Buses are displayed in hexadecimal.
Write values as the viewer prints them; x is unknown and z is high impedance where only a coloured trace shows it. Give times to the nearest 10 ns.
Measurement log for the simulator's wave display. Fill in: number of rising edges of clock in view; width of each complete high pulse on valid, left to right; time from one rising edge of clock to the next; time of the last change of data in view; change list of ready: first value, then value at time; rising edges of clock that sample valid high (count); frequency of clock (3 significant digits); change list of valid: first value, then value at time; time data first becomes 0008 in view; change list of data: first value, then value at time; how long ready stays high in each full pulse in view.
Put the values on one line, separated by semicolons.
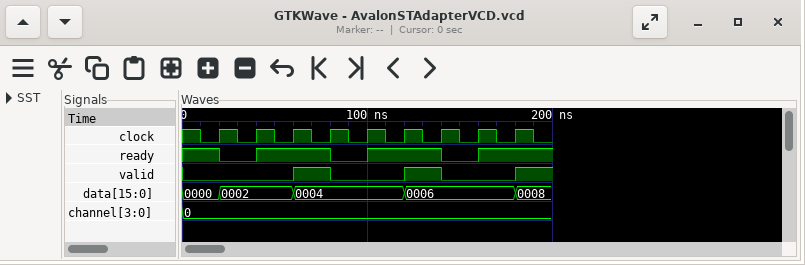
9; 20 ns, 20 ns; 20 ns; 180 ns; 1, 0 at 20 ns, 1 at 40 ns, 0 at 80 ns, 1 at 100 ns, 0 at 140 ns, 1 at 160 ns; 2; 50.0 MHz; 0, 1 at 60 ns, 0 at 80 ns, 1 at 120 ns, 0 at 140 ns, 1 at 180 ns; 180 ns; 0000, 0002 at 20 ns, 0004 at 60 ns, 0006 at 120 ns, 0008 at 180 ns; 40 ns, 40 ns
